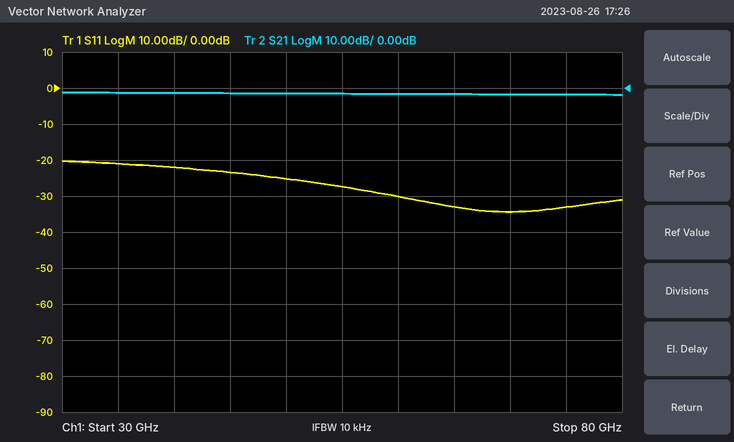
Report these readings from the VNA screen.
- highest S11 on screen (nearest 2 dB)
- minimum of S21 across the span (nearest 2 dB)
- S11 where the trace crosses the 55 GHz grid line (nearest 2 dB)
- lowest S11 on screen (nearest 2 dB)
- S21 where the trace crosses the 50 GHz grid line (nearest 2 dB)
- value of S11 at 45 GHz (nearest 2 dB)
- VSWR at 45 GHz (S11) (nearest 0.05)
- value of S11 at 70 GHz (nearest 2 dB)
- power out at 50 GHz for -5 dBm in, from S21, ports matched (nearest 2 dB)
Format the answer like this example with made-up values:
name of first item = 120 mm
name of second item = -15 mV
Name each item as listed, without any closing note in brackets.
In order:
highest S11 on screen = -20 dB
minimum of S21 across the span = -2 dB
S11 where the trace crosses the 55 GHz grid line = -28 dB
lowest S11 on screen = -34 dB
S21 where the trace crosses the 50 GHz grid line = -2 dB
value of S11 at 45 GHz = -24 dB
VSWR at 45 GHz (S11) = 1.15
value of S11 at 70 GHz = -34 dB
power out at 50 GHz for -5 dBm in, from S21, ports matched = -6 dBm
